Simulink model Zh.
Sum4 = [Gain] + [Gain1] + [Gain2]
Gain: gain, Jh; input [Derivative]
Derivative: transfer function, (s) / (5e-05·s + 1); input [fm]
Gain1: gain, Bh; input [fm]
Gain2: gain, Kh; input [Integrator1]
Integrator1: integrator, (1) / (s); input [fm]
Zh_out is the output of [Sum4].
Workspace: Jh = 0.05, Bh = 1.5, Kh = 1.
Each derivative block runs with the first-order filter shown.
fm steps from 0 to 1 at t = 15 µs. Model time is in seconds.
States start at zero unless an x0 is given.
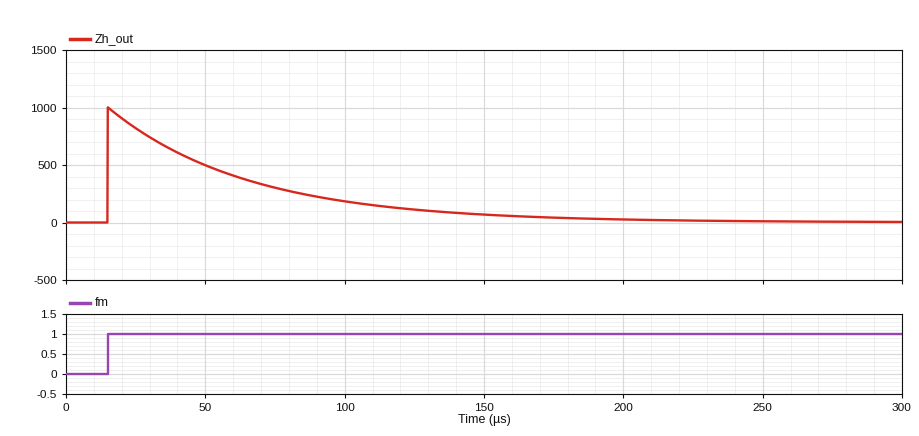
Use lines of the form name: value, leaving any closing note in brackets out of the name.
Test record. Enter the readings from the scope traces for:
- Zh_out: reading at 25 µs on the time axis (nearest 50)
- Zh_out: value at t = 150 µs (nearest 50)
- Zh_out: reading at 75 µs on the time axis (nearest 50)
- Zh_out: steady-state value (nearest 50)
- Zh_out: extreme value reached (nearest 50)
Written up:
Zh_out: reading at 25 µs on the time axis: 800
Zh_out: value at t = 150 µs: 50
Zh_out: reading at 75 µs on the time axis: 300
Zh_out: steady-state value: 0
Zh_out: extreme value reached: 1000
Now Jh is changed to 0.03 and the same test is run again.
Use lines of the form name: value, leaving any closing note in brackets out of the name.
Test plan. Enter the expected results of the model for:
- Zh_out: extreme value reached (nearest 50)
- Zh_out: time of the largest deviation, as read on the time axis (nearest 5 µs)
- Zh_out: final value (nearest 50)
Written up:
Zh_out: extreme value reached: 600
Zh_out: time of the largest deviation, as read on the time axis: 15 µs
Zh_out: final value: 0
